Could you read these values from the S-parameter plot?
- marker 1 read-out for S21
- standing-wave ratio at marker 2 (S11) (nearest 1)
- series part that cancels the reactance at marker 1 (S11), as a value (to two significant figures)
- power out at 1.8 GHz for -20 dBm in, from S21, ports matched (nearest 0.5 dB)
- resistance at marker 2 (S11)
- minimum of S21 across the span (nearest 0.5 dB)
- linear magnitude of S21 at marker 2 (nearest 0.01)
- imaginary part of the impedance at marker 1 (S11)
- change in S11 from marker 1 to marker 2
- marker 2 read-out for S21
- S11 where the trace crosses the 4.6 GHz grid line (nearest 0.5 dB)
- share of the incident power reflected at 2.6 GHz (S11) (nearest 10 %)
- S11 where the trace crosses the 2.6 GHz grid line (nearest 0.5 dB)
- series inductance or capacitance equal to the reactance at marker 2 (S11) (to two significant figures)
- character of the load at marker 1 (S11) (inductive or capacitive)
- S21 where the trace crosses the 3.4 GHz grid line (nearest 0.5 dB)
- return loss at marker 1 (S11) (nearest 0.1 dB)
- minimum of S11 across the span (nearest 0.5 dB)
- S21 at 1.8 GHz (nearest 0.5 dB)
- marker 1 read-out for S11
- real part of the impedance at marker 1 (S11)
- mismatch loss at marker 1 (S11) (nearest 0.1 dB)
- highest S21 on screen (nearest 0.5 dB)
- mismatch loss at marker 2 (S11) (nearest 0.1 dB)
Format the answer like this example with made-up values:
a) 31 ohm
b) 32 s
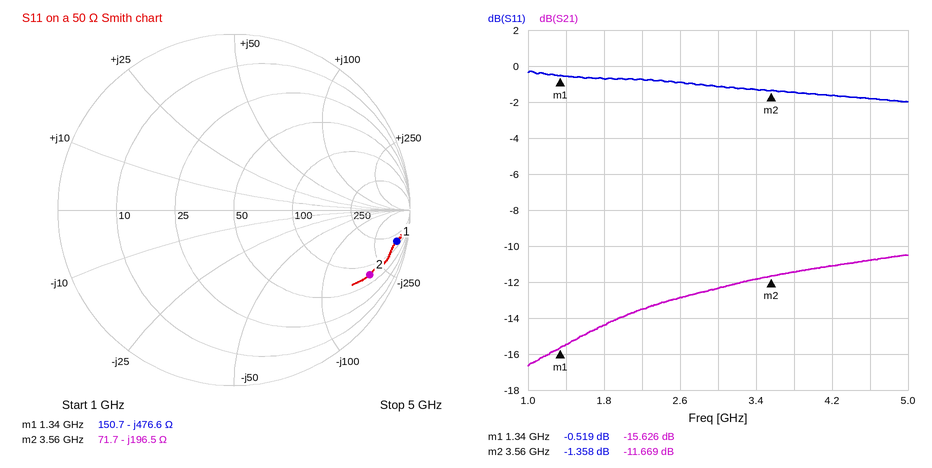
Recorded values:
a) -15.626 dB
b) 13
c) 57 nH
d) -34.5 dBm
e) 71.7 Ω
f) -16.5 dB
g) 0.26
h) -476.6 Ω
i) -0.839 dB
j) -11.669 dB
k) -2.0 dB
l) 80 %
m) -1.0 dB
n) 230 fF
o) capacitive
p) -12.0 dB
q) 0.5 dB
r) -2.0 dB
s) -14.5 dB
t) -0.519 dB
u) 150.7 Ω
v) 9.5 dB
w) -10.5 dB
x) 5.7 dB
